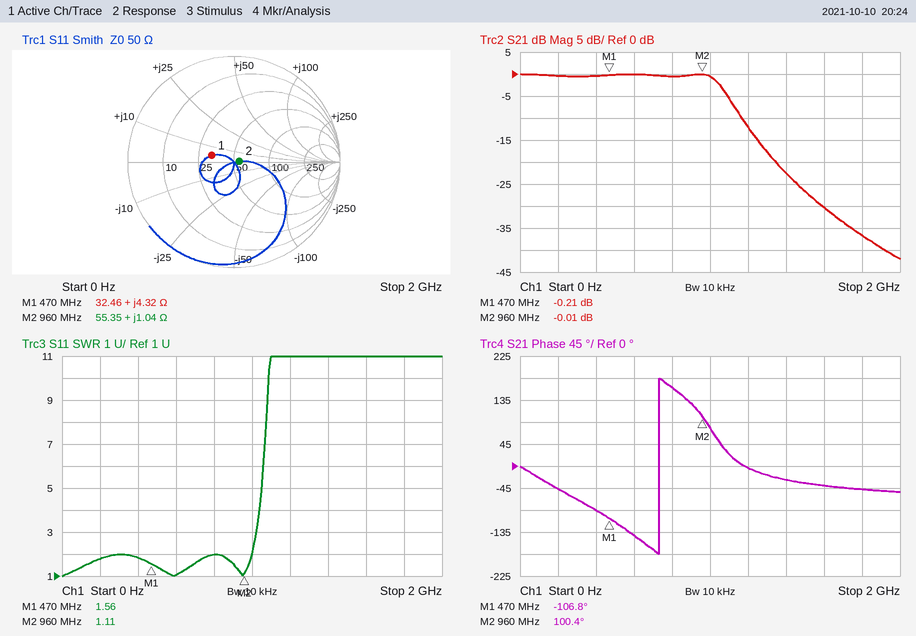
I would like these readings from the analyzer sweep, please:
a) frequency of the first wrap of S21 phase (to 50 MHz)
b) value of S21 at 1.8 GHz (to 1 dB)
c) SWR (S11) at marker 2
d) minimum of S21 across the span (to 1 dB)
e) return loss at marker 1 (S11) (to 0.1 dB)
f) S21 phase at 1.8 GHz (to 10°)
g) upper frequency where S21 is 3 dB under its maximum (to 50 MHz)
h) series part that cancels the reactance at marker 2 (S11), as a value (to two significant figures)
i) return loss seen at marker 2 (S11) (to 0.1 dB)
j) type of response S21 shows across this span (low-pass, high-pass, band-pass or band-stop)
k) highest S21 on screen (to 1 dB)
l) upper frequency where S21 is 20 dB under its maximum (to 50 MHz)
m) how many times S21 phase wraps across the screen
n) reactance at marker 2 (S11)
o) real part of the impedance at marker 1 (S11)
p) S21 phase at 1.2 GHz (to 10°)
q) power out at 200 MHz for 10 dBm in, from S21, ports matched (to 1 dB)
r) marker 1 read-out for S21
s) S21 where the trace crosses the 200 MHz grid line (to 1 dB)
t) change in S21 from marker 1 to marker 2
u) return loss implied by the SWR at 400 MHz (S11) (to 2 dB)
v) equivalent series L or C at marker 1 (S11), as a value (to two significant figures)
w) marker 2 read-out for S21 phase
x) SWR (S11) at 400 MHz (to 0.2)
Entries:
750 MHz
-37 dB
1.11
-42 dB
13.2 dB
-50°
1.05 GHz
160 pF
25.7 dB
low-pass
0 dB
1.35 GHz
1
+1.04 Ω
32.46 Ω
0°
10 dBm
-0.21 dB
0 dB
0.20 dB
10 dB
1.5 nH
100.4°
1.8
